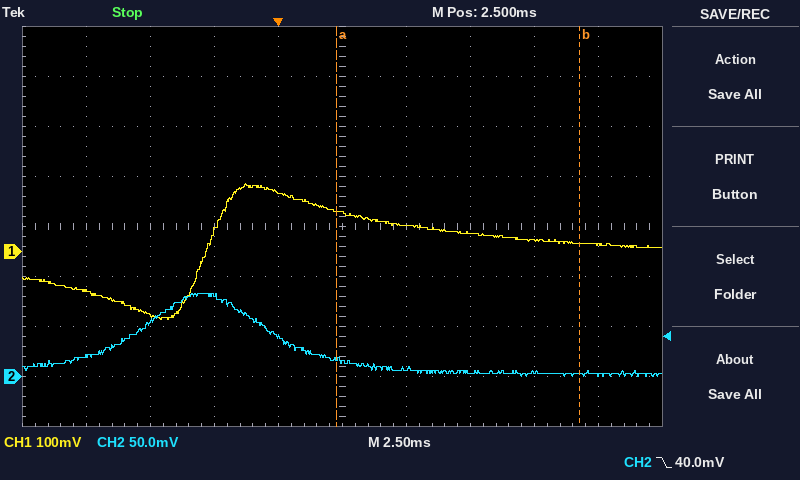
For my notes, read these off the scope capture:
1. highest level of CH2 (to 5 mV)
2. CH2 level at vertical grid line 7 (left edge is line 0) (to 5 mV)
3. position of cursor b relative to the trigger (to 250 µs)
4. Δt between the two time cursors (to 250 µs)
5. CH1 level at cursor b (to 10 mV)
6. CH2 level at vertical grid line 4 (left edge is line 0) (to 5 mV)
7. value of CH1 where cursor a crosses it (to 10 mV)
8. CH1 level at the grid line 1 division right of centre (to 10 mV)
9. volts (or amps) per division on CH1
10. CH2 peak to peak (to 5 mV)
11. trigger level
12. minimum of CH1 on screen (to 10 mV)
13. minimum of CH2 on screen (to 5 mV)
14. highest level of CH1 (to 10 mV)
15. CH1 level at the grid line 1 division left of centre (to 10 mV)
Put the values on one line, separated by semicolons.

85 mV; 5 mV; +11.75 ms; 9.50 ms; 20 mV; 40 mV; 80 mV; 50 mV; 100 mV; 85 mV; 40.0 mV; -140 mV; 0 mV; 140 mV; 120 mV
